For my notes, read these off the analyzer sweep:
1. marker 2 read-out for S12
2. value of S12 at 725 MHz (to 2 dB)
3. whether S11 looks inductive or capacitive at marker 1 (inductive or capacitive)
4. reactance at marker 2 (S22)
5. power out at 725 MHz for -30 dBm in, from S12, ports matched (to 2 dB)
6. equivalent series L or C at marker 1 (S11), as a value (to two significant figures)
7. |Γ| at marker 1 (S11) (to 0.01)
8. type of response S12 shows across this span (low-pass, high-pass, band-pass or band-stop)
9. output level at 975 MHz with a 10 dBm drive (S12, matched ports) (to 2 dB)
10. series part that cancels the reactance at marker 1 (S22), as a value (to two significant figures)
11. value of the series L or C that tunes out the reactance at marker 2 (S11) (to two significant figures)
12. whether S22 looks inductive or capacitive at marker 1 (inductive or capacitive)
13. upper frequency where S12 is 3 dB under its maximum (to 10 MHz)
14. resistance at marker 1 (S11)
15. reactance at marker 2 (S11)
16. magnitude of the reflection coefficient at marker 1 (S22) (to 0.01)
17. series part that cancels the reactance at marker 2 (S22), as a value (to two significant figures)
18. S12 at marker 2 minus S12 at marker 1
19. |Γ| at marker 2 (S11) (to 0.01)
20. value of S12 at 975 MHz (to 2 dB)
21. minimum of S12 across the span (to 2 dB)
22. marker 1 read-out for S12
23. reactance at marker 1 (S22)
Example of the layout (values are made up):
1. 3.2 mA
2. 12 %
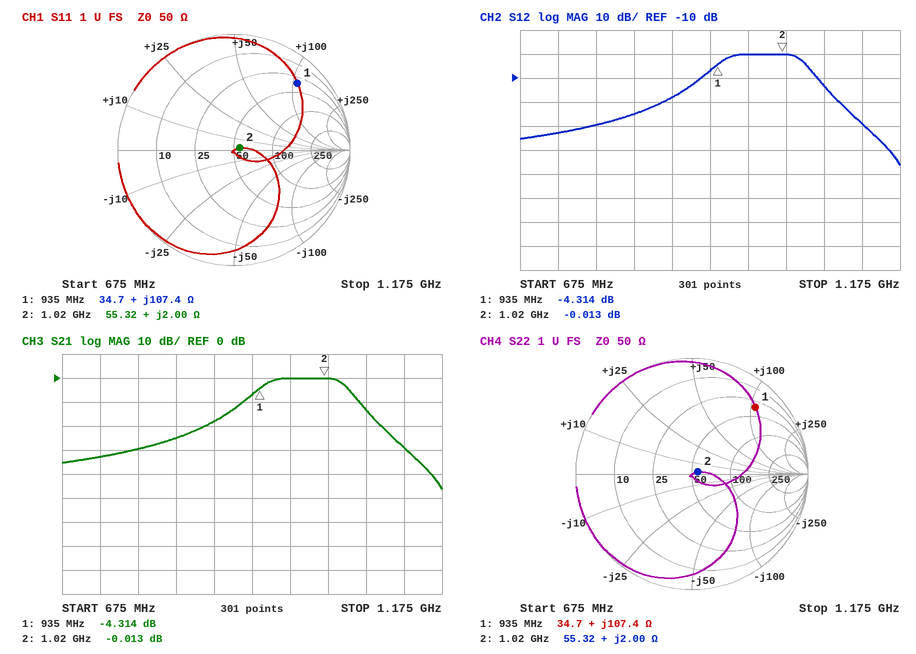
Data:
1. -0.013 dB
2. -32 dB
3. inductive
4. +2.00 Ω
5. -62 dBm
6. 18 nH
7. 0.79
8. band-pass
9. 10 dBm
10. 1.6 pF
11. 78 pF
12. inductive
13. 1.05 GHz
14. 34.7 Ω
15. +2.00 Ω
16. 0.79
17. 78 pF
18. 4.301 dB
19. 0.05
20. 0 dB
21. -46 dB
22. -4.314 dB
23. +107.4 Ω
